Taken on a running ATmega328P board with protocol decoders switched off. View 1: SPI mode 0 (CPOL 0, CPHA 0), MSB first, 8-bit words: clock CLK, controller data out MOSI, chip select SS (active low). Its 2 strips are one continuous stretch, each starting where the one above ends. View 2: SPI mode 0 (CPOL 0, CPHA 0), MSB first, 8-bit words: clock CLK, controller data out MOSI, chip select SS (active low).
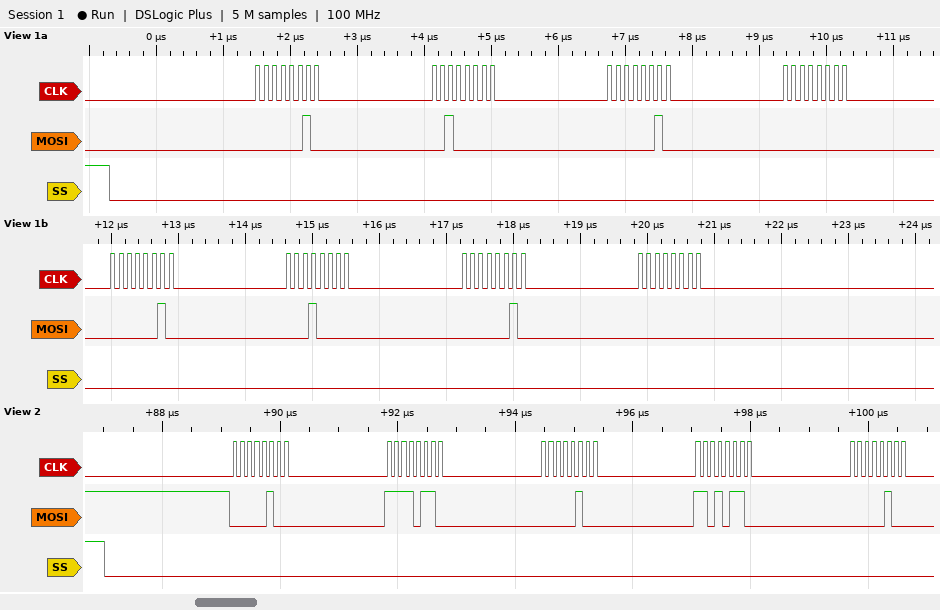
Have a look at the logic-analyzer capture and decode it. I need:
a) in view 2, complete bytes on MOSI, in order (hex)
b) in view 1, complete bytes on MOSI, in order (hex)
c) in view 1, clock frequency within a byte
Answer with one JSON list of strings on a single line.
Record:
["04 F6 04 D6 04", "02 20 02 00 02 10 02 00", "8 MHz"]
